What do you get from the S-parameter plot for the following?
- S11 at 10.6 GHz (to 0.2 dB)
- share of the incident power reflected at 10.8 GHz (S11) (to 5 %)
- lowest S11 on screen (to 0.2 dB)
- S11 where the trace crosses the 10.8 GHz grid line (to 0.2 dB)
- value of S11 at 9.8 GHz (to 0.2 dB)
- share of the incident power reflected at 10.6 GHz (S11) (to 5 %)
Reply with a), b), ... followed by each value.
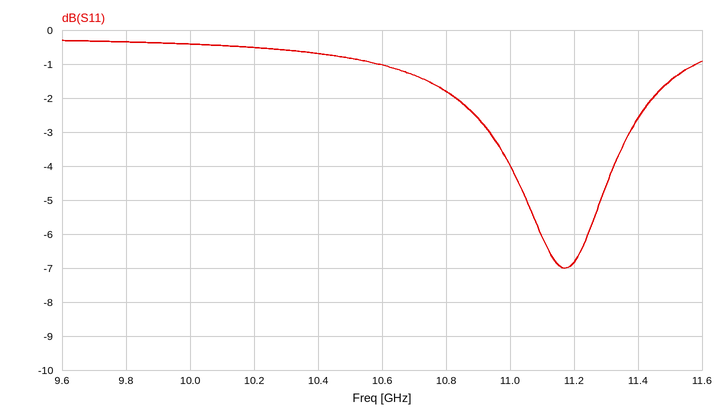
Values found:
a) -1.0 dB
b) 65 %
c) -7.0 dB
d) -1.8 dB
e) -0.4 dB
f) 80 %
